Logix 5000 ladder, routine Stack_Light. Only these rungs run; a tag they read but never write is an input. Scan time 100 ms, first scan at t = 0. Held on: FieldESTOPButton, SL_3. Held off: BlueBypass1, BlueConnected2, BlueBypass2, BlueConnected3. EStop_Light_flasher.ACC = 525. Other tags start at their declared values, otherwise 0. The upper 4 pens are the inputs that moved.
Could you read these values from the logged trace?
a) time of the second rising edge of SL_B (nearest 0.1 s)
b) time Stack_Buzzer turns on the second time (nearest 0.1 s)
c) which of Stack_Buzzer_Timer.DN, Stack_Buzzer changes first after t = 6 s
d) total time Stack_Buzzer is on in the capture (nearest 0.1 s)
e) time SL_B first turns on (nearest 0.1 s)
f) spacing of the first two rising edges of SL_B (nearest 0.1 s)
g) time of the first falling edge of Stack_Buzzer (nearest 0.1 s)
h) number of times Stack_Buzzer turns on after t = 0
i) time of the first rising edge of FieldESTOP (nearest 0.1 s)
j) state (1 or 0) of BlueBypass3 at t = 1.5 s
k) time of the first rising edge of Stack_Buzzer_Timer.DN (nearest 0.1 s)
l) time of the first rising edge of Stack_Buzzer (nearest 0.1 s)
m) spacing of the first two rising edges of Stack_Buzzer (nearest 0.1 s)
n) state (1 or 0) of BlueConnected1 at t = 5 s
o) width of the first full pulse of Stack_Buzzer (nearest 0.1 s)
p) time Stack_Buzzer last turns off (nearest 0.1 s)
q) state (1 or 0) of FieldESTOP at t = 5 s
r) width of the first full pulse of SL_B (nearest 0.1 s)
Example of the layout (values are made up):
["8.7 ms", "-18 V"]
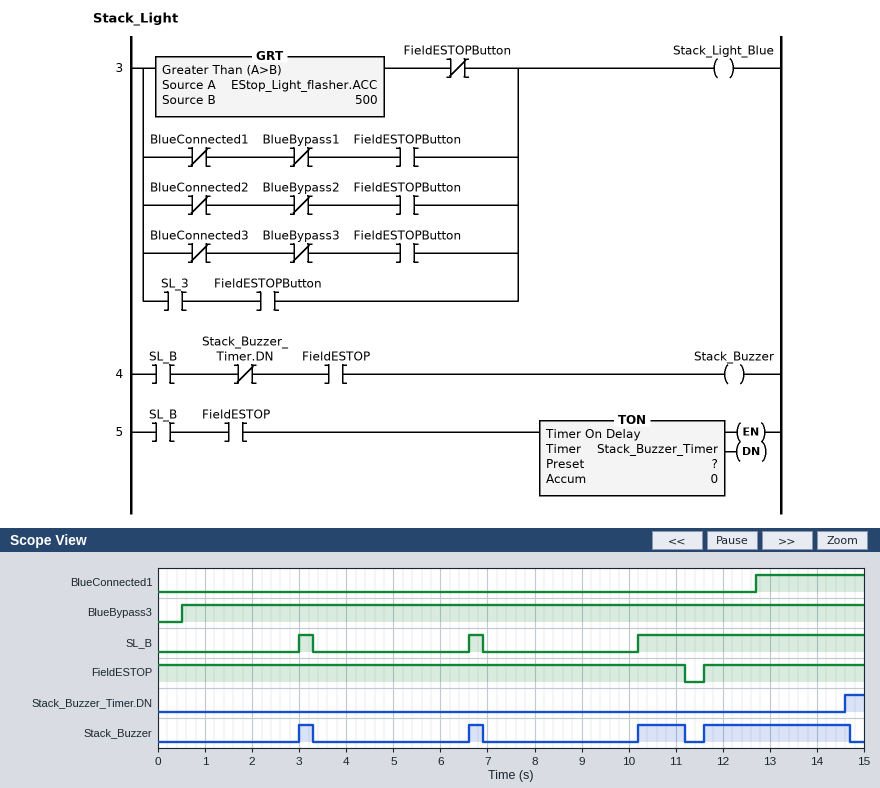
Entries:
["6.6 s", "6.6 s", "Stack_Buzzer", "4.7 s", "3.0 s", "3.6 s", "3.3 s", "4", "11.6 s", "1", "14.6 s", "3.0 s", "3.6 s", "0", "0.3 s", "14.7 s", "1", "0.3 s"]
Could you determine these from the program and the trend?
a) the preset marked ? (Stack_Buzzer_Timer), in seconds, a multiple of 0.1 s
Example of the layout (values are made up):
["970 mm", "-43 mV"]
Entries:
["3.0 s"]
